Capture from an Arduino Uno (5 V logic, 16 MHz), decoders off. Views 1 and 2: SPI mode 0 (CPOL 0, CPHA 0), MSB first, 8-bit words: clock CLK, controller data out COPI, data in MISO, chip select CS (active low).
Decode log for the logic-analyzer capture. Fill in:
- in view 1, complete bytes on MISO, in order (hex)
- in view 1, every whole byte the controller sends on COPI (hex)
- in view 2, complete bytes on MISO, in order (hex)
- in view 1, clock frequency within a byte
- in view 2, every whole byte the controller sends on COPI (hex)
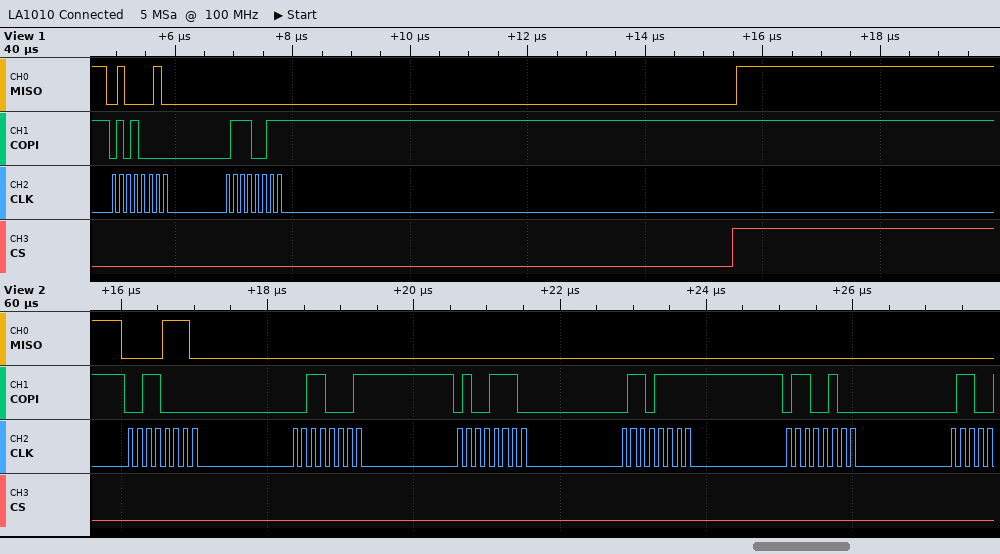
0x42 0x00
0x50 0x73
0x0E 0x00 0x00 0x00 0x00
8 MHz
0x30 0x31 0x4E 0x6F 0x64
